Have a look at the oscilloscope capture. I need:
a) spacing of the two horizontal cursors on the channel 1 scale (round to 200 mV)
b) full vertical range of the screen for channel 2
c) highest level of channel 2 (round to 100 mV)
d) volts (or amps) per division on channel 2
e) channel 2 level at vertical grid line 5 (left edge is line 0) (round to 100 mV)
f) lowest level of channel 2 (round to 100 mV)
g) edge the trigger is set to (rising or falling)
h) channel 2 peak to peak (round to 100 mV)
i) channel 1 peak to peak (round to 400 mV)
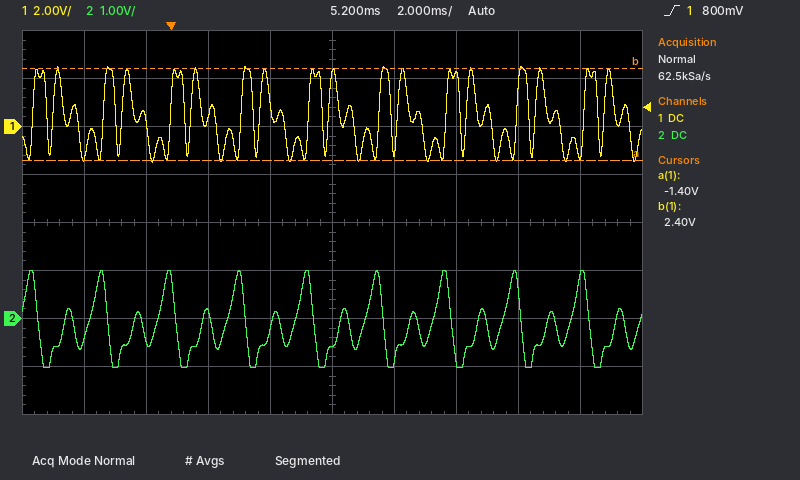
3.8 V
8 V
1.0 V
1 V
-600 mV
-1.0 V
rising
2.0 V
4.0 V
